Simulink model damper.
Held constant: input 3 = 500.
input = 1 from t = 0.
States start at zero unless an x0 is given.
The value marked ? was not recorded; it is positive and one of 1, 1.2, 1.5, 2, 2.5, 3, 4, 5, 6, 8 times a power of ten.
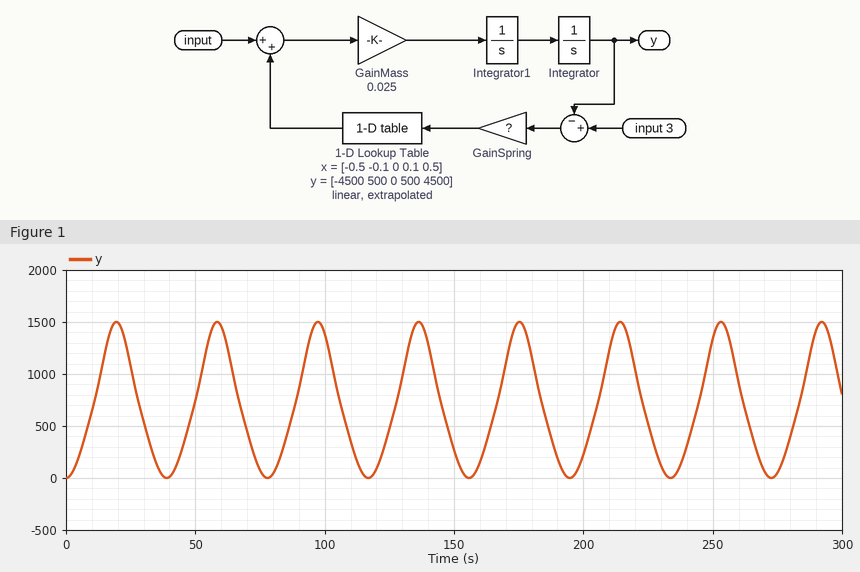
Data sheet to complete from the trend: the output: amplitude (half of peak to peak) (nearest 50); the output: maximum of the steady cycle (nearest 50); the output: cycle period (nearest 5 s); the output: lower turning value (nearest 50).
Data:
750
1500
40 s
0
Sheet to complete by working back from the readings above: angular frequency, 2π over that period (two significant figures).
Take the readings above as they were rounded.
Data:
0.16 rad/s
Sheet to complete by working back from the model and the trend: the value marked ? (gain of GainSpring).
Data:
0.00025
